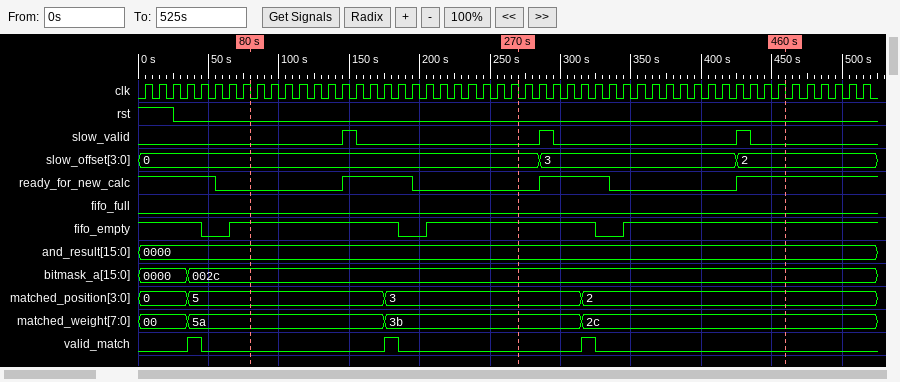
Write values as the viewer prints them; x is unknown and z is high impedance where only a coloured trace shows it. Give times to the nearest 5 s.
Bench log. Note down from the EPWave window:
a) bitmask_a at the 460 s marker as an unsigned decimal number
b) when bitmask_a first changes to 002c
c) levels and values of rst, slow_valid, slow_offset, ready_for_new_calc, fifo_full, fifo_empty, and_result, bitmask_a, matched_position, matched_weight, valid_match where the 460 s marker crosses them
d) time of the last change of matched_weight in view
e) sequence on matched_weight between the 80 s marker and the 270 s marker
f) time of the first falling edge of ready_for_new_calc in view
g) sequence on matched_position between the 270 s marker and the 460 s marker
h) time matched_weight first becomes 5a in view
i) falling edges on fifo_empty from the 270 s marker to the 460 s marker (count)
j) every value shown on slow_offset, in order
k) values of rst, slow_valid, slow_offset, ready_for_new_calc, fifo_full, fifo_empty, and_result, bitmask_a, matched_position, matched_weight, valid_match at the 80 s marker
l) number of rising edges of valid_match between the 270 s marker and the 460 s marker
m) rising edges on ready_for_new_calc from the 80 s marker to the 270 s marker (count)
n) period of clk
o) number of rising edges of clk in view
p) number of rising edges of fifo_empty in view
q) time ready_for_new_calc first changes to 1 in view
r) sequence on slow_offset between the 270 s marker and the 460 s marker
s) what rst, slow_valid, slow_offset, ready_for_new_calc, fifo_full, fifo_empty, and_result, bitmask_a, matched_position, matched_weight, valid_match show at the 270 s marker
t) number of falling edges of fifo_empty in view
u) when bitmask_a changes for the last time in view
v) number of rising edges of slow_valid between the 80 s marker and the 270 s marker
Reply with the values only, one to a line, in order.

44
35 s
rst=0, slow_valid=0, slow_offset=2, ready_for_new_calc=1, fifo_full=0, fifo_empty=1, and_result=0000, bitmask_a=002c, matched_position=2, matched_weight=2c, valid_match=0
315 s
5a, 3b
55 s
3, 2
35 s
1
0, 3, 2
rst=0, slow_valid=0, slow_offset=0, ready_for_new_calc=0, fifo_full=0, fifo_empty=1, and_result=0000, bitmask_a=002c, matched_position=5, matched_weight=5a, valid_match=0
1
1
10 s
52
3
145 s
0, 3, 2
rst=0, slow_valid=0, slow_offset=0, ready_for_new_calc=0, fifo_full=0, fifo_empty=1, and_result=0000, bitmask_a=002c, matched_position=3, matched_weight=3b, valid_match=0
3
35 s
1
